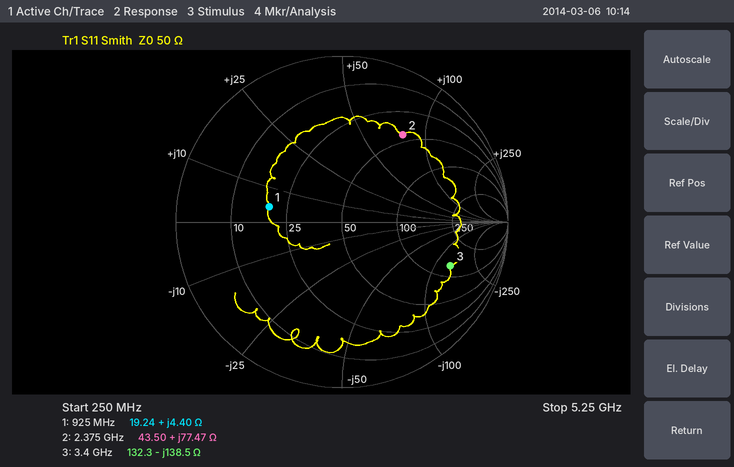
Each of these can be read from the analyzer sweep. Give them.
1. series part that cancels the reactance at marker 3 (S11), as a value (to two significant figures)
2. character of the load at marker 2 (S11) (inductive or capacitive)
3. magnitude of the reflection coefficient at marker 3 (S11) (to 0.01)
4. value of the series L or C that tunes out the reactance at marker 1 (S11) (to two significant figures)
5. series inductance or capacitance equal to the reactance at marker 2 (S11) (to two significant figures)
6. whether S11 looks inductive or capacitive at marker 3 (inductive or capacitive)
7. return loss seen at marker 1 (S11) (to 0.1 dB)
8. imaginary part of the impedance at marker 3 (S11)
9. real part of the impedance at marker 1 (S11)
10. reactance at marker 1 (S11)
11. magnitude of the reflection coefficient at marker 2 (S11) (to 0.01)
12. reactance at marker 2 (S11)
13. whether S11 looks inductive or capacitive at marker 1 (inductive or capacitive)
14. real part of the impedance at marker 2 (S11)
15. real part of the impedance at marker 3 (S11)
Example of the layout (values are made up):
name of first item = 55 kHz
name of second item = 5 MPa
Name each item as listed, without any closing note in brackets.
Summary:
series part that cancels the reactance at marker 3 (S11), as a value = 6.5 nH
character of the load at marker 2 (S11) = inductive
magnitude of the reflection coefficient at marker 3 (S11) = 0.70
value of the series L or C that tunes out the reactance at marker 1 (S11) = 39 pF
series inductance or capacitance equal to the reactance at marker 2 (S11) = 5.2 nH
whether S11 looks inductive or capacitive at marker 3 = capacitive
return loss seen at marker 1 (S11) = 7.0 dB
imaginary part of the impedance at marker 3 = -138.5 Ω
real part of the impedance at marker 1 = 19.24 Ω
reactance at marker 1 = +4.40 Ω
magnitude of the reflection coefficient at marker 2 (S11) = 0.64
reactance at marker 2 = +77.47 Ω
whether S11 looks inductive or capacitive at marker 1 = inductive
real part of the impedance at marker 2 = 43.50 Ω
real part of the impedance at marker 3 = 132.3 Ω
